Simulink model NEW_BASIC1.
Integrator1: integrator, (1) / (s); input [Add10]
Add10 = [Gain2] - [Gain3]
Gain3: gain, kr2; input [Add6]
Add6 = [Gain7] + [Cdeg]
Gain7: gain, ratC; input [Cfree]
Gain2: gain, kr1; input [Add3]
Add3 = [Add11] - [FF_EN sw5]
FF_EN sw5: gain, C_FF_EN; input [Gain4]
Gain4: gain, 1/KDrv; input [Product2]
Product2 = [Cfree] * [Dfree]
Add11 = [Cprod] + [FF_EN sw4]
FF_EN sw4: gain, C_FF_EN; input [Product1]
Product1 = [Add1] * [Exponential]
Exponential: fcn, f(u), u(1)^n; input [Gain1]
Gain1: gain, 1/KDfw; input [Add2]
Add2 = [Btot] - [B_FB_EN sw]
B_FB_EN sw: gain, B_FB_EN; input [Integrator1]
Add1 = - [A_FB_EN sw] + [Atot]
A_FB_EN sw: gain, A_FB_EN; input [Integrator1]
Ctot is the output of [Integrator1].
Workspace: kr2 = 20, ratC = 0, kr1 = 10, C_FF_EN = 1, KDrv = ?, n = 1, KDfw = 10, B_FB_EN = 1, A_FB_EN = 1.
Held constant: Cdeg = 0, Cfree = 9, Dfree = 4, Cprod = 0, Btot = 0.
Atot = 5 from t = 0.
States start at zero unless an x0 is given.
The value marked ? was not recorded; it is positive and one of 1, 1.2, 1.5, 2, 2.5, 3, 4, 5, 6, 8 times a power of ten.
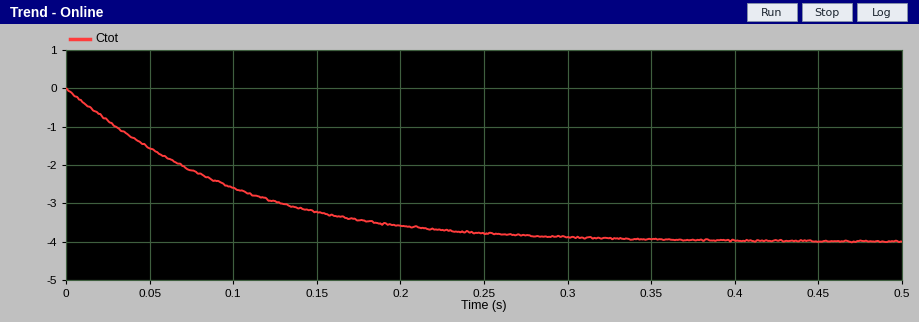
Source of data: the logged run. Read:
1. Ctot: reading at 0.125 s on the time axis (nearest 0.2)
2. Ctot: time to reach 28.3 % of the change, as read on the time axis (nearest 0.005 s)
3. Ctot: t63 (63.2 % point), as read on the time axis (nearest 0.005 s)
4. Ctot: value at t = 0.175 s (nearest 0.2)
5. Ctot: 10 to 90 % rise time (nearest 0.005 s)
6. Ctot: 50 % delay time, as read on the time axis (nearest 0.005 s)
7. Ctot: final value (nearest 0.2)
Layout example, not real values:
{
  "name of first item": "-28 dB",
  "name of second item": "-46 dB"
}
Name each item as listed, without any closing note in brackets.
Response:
{
  "Ctot: reading at 0.125 s on the time axis": "-3.0",
  "Ctot: time to reach 28.3 % of the change, as read on the time axis": "0.035 s",
  "Ctot: t63 (63.2 % point), as read on the time axis": "0.095 s",
  "Ctot: value at t = 0.175 s": "-3.4",
  "Ctot: 10 to 90 % rise time": "0.190 s",
  "Ctot: 50 % delay time, as read on the time axis": "0.070 s",
  "Ctot: final value": "-4.0"
}
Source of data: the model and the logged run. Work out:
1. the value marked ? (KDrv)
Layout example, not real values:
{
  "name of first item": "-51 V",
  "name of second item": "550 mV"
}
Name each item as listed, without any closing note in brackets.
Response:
{
  "the value marked ?": "10"
}
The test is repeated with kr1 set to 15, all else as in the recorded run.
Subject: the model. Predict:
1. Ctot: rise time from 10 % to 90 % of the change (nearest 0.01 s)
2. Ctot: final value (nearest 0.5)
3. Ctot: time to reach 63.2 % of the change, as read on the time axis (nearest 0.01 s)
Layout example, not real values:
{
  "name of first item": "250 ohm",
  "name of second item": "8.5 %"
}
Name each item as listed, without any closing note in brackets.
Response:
{
  "Ctot: rise time from 10 % to 90 % of the change": "0.13 s",
  "Ctot: final value": "-4.0",
  "Ctot: time to reach 63.2 % of the change, as read on the time axis": "0.06 s"
}
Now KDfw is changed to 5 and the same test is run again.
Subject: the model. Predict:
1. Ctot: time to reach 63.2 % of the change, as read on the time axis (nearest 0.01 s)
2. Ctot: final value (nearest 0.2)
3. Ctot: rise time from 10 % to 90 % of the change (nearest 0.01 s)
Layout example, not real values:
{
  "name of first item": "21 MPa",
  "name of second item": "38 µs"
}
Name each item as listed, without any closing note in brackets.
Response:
{
  "Ctot: time to reach 63.2 % of the change, as read on the time axis": "0.06 s",
  "Ctot: final value": "-2.4",
  "Ctot: rise time from 10 % to 90 % of the change": "0.12 s"
}
